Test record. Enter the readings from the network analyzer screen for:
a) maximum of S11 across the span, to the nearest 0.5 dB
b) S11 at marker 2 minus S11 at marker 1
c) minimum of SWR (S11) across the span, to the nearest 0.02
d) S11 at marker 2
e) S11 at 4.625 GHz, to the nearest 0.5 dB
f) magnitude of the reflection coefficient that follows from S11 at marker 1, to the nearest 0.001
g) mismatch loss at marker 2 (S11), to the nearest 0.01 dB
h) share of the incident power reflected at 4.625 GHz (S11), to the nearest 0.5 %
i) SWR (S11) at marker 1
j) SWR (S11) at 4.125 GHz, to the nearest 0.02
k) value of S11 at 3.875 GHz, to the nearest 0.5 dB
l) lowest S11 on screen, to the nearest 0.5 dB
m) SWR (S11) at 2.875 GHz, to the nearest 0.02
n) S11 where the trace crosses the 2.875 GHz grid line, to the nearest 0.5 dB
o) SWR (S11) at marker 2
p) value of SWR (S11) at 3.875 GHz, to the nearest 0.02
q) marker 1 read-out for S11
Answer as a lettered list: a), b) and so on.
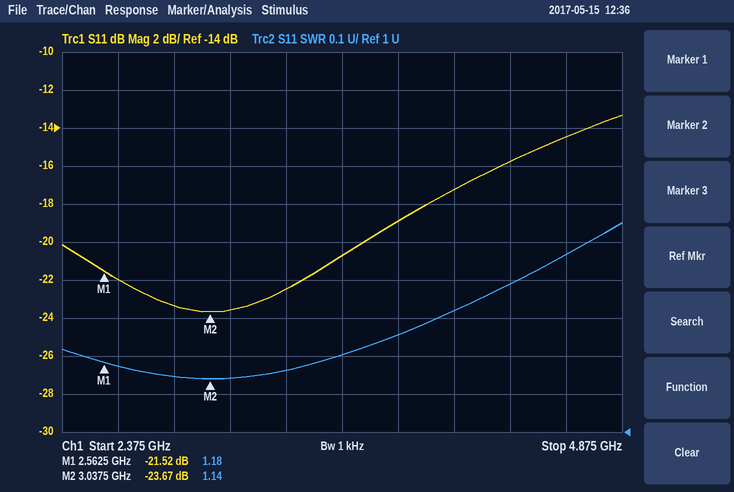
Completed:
a) -13.5 dB
b) -2.15 dB
c) 1.14
d) -23.67 dB
e) -14.5 dB
f) 0.084
g) 0.02 dB
h) 3.5 %
i) 1.18
j) 1.32
k) -19.0 dB
l) -23.5 dB
m) 1.14
n) -23.5 dB
o) 1.14
p) 1.26
q) -21.52 dB
